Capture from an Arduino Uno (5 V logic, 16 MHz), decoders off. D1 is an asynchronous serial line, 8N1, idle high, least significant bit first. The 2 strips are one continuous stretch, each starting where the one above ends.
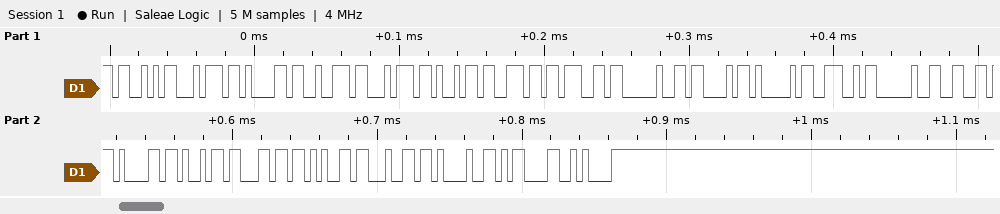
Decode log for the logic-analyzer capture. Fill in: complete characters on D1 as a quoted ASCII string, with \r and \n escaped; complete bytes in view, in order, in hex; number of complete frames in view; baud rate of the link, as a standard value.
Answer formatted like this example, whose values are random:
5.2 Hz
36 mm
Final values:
"Starting CAN failed!\r\n"
53 74 61 72 74 69 6E 67 20 43 41 4E 20 66 61 69 6C 65 64 21 0D 0A
22
250000 baud
